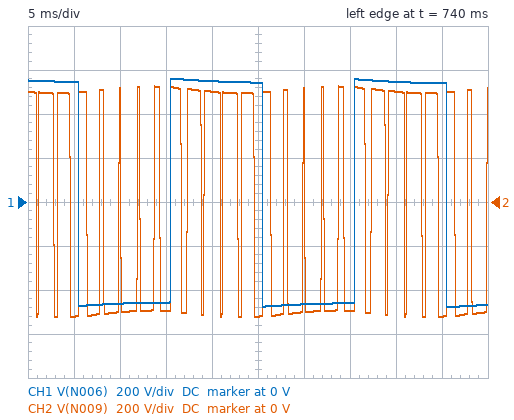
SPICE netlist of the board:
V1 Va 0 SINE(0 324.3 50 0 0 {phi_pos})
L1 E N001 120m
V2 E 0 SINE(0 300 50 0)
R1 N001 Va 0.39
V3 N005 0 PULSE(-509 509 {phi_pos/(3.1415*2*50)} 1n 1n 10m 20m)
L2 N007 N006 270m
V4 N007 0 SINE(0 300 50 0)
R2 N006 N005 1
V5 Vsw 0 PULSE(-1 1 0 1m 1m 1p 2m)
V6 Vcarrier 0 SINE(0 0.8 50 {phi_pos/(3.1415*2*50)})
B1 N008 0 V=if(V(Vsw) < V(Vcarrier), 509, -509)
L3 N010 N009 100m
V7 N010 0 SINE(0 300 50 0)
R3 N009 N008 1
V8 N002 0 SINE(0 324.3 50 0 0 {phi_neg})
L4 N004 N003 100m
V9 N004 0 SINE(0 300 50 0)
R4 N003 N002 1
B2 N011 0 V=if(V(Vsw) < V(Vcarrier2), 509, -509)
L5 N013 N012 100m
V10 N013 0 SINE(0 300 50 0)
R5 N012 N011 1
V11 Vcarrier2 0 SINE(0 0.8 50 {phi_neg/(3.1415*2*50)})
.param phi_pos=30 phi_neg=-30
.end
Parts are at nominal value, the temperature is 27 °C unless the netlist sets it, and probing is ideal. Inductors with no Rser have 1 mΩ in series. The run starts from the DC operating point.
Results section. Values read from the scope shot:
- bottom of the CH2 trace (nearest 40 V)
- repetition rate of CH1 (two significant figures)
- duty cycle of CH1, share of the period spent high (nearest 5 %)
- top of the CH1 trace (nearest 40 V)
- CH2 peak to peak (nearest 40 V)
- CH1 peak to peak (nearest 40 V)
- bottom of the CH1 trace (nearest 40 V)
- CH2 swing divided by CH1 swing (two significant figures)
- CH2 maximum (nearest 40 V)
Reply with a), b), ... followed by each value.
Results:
a) -520 V
b) 50 Hz
c) 50 %
d) 560 V
e) 1.04 kV
f) 1.04 kV
g) -480 V
h) 1.0
i) 520 V
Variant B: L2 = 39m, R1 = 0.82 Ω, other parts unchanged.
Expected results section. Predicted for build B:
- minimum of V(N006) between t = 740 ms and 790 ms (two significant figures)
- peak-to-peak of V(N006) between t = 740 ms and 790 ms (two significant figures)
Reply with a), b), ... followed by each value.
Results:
a) -570 V
b) 1.1 kV
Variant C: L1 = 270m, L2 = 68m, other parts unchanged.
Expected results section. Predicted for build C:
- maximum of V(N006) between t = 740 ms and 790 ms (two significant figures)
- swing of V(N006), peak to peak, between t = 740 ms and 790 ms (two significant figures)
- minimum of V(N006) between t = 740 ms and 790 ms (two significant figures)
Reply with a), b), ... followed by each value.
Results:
a) 540 V
b) 1.1 kV
c) -540 V
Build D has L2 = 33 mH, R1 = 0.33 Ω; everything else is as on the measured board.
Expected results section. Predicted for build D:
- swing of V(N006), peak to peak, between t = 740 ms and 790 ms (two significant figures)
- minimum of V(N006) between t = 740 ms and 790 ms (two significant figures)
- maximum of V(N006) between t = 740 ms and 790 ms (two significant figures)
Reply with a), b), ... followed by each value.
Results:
a) 1.2 kV
b) -580 V
c) 580 V
